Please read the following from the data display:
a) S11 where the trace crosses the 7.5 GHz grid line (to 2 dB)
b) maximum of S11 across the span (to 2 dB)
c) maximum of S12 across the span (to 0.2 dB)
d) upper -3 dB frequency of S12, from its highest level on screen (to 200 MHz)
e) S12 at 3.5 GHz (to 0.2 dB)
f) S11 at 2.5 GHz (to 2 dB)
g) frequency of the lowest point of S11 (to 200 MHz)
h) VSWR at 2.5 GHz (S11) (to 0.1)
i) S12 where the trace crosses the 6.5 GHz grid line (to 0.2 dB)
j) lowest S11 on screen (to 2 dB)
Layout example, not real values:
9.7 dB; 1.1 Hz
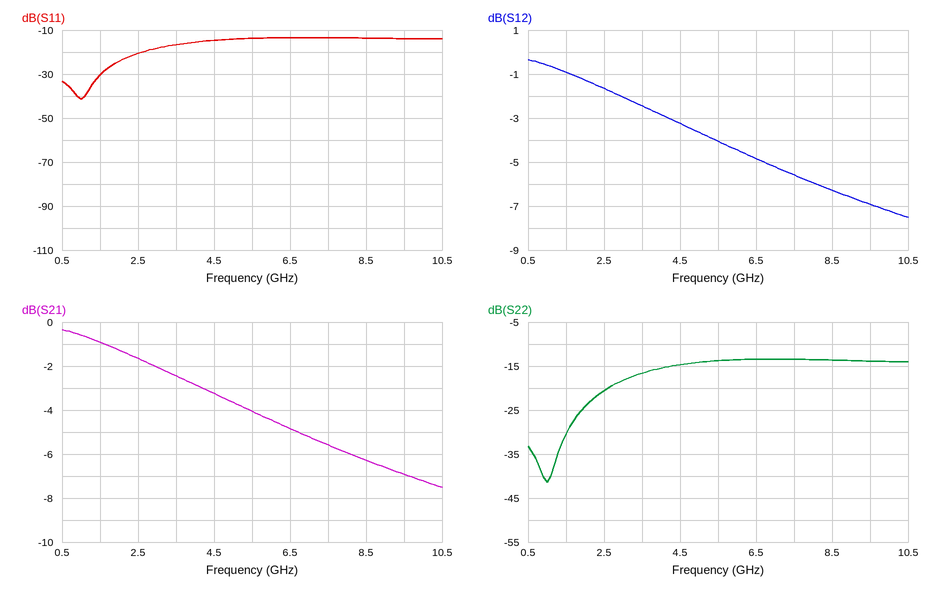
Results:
-14 dB; -14 dB; -0.4 dB; 4.6 GHz; -2.4 dB; -20 dB; 1.0 GHz; 1.2; -4.8 dB; -42 dB
